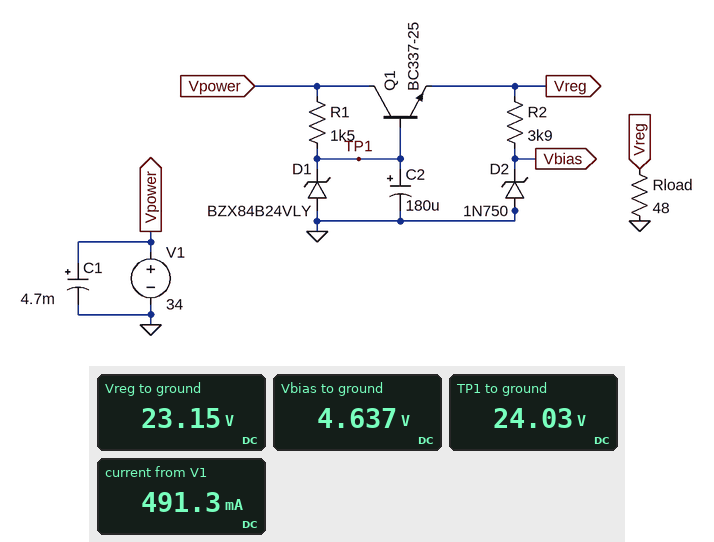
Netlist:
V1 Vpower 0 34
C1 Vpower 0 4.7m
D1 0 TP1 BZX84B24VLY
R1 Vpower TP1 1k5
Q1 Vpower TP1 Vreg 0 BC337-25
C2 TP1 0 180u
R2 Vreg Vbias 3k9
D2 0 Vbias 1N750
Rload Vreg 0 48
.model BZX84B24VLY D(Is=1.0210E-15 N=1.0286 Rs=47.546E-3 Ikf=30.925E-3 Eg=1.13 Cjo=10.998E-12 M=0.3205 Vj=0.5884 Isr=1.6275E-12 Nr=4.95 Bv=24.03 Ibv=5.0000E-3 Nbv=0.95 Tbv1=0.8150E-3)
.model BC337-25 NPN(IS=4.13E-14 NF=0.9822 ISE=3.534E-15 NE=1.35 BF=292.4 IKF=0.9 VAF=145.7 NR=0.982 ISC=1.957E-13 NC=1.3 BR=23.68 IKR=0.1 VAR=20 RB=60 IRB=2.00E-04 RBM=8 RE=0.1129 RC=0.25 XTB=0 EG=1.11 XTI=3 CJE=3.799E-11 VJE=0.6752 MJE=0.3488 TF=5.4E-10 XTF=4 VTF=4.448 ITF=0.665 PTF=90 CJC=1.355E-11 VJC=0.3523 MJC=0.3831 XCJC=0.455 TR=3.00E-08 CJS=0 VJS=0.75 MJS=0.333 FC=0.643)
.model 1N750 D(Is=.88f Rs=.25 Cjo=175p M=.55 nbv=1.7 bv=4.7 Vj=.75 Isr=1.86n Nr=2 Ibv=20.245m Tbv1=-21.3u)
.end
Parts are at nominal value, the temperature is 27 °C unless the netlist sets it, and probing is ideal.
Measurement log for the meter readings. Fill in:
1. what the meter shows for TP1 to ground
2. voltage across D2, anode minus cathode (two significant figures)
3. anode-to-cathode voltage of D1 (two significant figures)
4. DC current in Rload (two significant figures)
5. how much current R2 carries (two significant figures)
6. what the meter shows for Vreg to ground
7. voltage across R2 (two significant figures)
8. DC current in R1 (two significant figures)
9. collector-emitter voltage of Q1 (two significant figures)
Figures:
24.03 V
-4.6 V
-24 V
480 mA
4.7 mA
23.15 V
19 V
6.6 mA
11 V
